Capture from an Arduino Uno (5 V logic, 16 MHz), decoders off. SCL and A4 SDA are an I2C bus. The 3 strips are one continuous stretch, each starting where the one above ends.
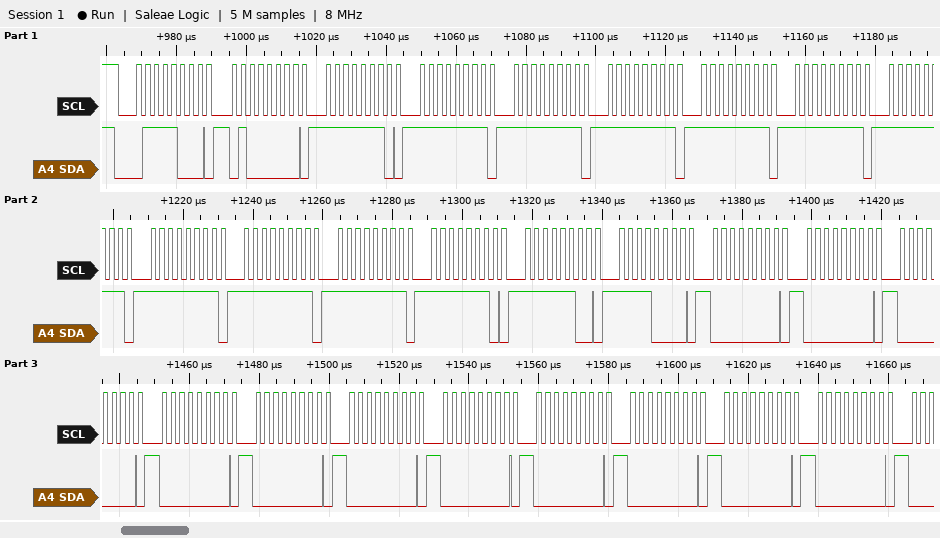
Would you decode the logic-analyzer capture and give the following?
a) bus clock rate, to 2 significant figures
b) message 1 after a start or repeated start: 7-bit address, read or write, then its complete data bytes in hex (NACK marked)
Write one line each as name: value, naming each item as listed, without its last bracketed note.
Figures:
bus clock rate, to 2 significant figures: 400 kHz
message 1 after a start or repeated start: 7-bit address, read or write, then its complete data bytes in hex: 0x3C write: 40 FE FF FF FF FF FF FF FF FF FF FE FC F0 00 00 00 00 00 00 00 00 00 00 00
